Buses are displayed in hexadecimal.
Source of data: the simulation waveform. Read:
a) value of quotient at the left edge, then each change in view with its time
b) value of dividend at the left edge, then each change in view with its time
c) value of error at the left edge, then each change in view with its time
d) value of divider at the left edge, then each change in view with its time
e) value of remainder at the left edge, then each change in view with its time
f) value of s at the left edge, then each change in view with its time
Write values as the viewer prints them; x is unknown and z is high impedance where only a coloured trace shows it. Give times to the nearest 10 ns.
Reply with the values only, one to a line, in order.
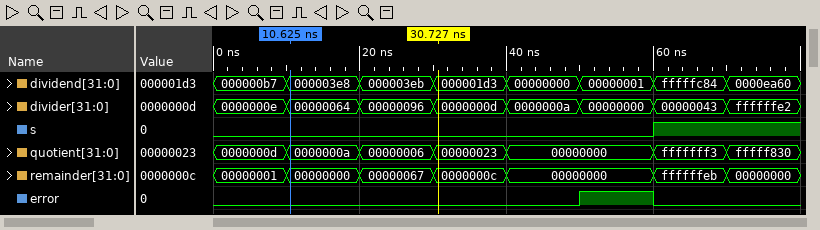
0000000d, 0000000a at 10 ns, 00000006 at 20 ns, 00000023 at 30 ns, 00000000 at 40 ns, fffffff3 at 60 ns, fffff830 at 70 ns
000000b7, 000003e8 at 10 ns, 000003eb at 20 ns, 000001d3 at 30 ns, 00000000 at 40 ns, 00000001 at 50 ns, fffffc84 at 60 ns, 0000ea60 at 70 ns
0, 1 at 50 ns, 0 at 60 ns
0000000e, 00000064 at 10 ns, 00000096 at 20 ns, 0000000d at 30 ns, 0000000a at 40 ns, 00000000 at 50 ns, 00000043 at 60 ns, ffffffe2 at 70 ns
00000001, 00000000 at 10 ns, 00000067 at 20 ns, 0000000c at 30 ns, 00000000 at 40 ns, ffffffeb at 60 ns, 00000000 at 70 ns
0, 1 at 60 ns
